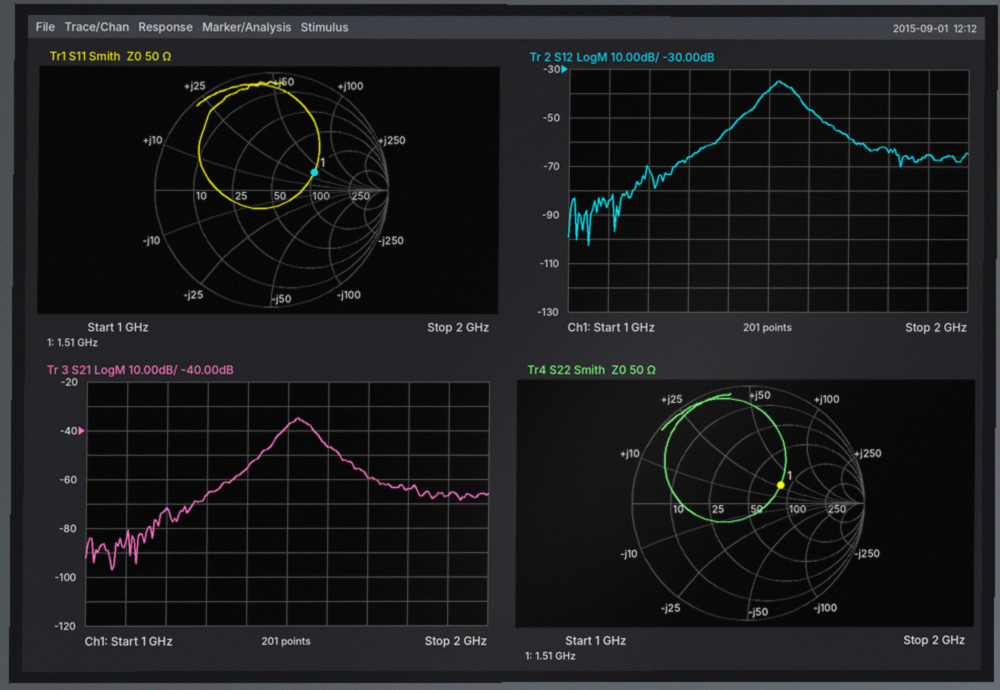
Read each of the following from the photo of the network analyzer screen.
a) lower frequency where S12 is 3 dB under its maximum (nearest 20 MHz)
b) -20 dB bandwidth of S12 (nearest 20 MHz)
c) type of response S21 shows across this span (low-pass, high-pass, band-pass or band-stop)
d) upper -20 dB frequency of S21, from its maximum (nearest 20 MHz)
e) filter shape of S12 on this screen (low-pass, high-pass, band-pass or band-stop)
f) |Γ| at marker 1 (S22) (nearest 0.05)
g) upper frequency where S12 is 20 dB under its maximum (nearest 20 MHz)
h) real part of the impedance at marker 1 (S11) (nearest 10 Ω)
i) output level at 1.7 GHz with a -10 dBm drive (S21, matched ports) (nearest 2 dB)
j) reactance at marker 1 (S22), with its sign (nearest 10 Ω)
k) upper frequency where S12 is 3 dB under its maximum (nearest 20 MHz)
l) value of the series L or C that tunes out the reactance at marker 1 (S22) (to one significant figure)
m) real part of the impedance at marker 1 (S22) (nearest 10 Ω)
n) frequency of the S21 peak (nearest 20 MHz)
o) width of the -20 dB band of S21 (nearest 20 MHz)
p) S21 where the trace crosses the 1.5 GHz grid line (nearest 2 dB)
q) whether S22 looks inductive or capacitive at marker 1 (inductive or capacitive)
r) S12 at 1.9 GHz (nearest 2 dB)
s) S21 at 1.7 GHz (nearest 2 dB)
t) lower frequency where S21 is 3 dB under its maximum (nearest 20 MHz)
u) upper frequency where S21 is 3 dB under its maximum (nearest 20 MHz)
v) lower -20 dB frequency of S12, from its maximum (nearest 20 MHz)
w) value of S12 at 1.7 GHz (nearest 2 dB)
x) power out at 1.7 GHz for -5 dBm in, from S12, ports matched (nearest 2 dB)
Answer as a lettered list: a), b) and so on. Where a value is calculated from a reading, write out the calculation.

a) 1.50 GHz
b) 1.66 GHz − 1.40 GHz = 260 MHz
c) band-pass
d) 1.66 GHz
e) band-pass
f) 0.30
g) 1.66 GHz
h) 100 Ω
i) -10 dBm + (-60 dB) = -70 dBm
j) +30 Ω
k) 1.56 GHz
l) C = 1/(2π × 1.51 GHz × 30 Ω) ≈ 4 pF
m) 80 Ω
n) 1.52 GHz
o) 1.66 GHz − 1.40 GHz = 260 MHz
p) -38 dB
q) inductive
r) -66 dB
s) -60 dB
t) 1.50 GHz
u) 1.56 GHz
v) 1.40 GHz
w) -58 dB
x) -5 dBm + (-58 dB) = -64 dBm
